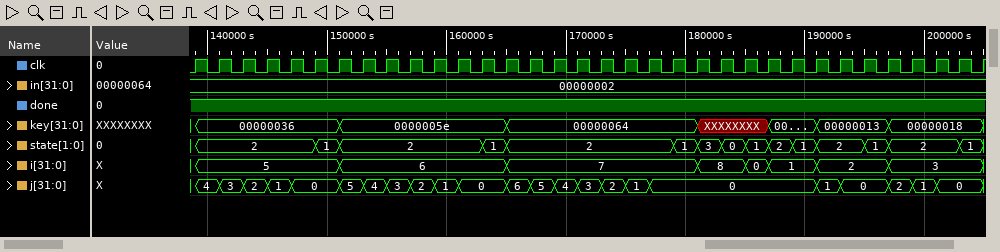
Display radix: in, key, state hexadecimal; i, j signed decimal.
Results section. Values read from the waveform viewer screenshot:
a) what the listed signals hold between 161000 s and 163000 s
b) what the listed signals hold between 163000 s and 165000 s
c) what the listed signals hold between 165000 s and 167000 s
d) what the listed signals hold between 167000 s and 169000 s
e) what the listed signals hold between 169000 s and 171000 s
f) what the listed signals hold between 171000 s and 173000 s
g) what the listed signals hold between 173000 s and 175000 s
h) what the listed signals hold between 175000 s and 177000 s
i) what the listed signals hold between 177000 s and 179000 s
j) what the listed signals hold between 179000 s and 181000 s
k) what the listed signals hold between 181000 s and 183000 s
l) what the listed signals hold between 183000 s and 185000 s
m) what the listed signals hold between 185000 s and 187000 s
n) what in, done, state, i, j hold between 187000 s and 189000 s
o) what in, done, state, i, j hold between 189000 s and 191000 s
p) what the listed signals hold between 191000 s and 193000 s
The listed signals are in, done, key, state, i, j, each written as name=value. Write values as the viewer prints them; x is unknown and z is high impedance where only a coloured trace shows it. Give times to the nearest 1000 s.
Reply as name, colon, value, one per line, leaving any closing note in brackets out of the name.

what the listed signals hold between 161000 s and 163000 s: in=00000002, done=1, key=0000005e, state=2, i=6, j=0
what the listed signals hold between 163000 s and 165000 s: in=00000002, done=1, key=0000005e, state=1, i=6, j=0
what the listed signals hold between 165000 s and 167000 s: in=00000002, done=1, key=00000064, state=2, i=7, j=6
what the listed signals hold between 167000 s and 169000 s: in=00000002, done=1, key=00000064, state=2, i=7, j=5
what the listed signals hold between 169000 s and 171000 s: in=00000002, done=1, key=00000064, state=2, i=7, j=4
what the listed signals hold between 171000 s and 173000 s: in=00000002, done=1, key=00000064, state=2, i=7, j=3
what the listed signals hold between 173000 s and 175000 s: in=00000002, done=1, key=00000064, state=2, i=7, j=2
what the listed signals hold between 175000 s and 177000 s: in=00000002, done=1, key=00000064, state=2, i=7, j=1
what the listed signals hold between 177000 s and 179000 s: in=00000002, done=1, key=00000064, state=2, i=7, j=0
what the listed signals hold between 179000 s and 181000 s: in=00000002, done=1, key=00000064, state=1, i=7, j=0
what the listed signals hold between 181000 s and 183000 s: in=00000002, done=1, key=XXXXXXXX, state=3, i=8, j=0
what the listed signals hold between 183000 s and 185000 s: in=00000002, done=1, key=XXXXXXXX, state=0, i=8, j=0
what the listed signals hold between 185000 s and 187000 s: in=00000002, done=1, key=XXXXXXXX, state=1, i=0, j=0
what in, done, state, i, j hold between 187000 s and 189000 s: in=00000002, done=1, state=2, i=1, j=0
what in, done, state, i, j hold between 189000 s and 191000 s: in=00000002, done=1, state=1, i=1, j=0
what the listed signals hold between 191000 s and 193000 s: in=00000002, done=1, key=00000013, state=2, i=2, j=1
